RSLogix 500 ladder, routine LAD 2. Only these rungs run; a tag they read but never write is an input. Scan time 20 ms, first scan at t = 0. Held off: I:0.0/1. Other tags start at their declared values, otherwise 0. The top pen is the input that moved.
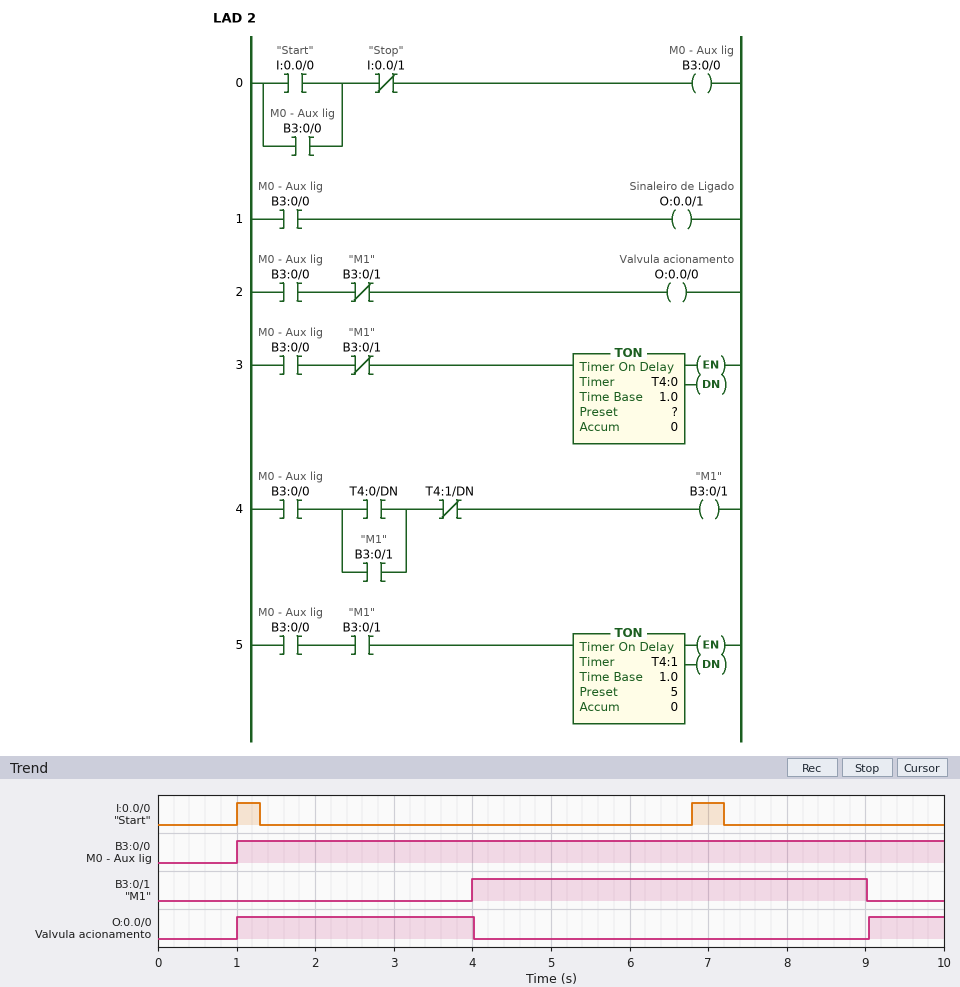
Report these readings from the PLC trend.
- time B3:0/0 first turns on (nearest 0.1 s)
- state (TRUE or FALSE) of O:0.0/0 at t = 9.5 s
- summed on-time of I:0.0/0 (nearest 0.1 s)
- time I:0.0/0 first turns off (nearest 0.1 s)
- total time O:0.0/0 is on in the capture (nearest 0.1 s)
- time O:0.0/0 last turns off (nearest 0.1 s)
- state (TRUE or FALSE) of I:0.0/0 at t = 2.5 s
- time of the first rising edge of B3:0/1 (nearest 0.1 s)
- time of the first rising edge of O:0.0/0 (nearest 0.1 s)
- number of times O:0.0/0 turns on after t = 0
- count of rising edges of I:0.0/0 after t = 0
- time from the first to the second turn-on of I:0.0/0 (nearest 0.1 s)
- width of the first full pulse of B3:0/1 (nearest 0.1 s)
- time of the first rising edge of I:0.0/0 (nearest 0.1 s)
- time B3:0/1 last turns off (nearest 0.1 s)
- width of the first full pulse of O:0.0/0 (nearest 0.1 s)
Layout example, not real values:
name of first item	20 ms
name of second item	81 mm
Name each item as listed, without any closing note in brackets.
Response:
time B3:0/0 first turns on	1.0 s
state (TRUE or FALSE) of O:0.0/0 at t = 9.5 s	TRUE
summed on-time of I:0.0/0	0.7 s
time I:0.0/0 first turns off	1.3 s
total time O:0.0/0 is on in the capture	4.0 s
time O:0.0/0 last turns off	4.0 s
state (TRUE or FALSE) of I:0.0/0 at t = 2.5 s	FALSE
time of the first rising edge of B3:0/1	4.0 s
time of the first rising edge of O:0.0/0	1.0 s
number of times O:0.0/0 turns on after t = 0	2
count of rising edges of I:0.0/0 after t = 0	2
time from the first to the second turn-on of I:0.0/0	5.8 s
width of the first full pulse of B3:0/1	5.0 s
time of the first rising edge of I:0.0/0	1.0 s
time B3:0/1 last turns off	9.0 s
width of the first full pulse of O:0.0/0	3.0 s
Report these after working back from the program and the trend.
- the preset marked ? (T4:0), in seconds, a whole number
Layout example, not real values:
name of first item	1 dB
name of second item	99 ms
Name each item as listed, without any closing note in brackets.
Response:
the preset marked ? (T4:0), in seconds, a whole number	3 s
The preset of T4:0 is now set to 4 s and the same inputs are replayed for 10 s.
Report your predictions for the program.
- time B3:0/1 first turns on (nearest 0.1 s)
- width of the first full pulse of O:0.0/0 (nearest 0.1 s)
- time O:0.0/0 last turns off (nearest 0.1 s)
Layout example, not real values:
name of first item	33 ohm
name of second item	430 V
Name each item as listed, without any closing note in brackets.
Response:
time B3:0/1 first turns on	5.0 s
width of the first full pulse of O:0.0/0	4.0 s
time O:0.0/0 last turns off	5.0 s
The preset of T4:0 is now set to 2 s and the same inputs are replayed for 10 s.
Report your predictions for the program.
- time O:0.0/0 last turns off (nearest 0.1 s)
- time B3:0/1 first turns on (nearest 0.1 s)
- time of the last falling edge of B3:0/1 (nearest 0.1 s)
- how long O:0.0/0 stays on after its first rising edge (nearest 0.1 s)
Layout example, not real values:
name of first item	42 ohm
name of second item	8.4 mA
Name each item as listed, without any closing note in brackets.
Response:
time O:0.0/0 last turns off	3.0 s
time B3:0/1 first turns on	3.0 s
time of the last falling edge of B3:0/1	8.0 s
how long O:0.0/0 stays on after its first rising edge	2.0 s
